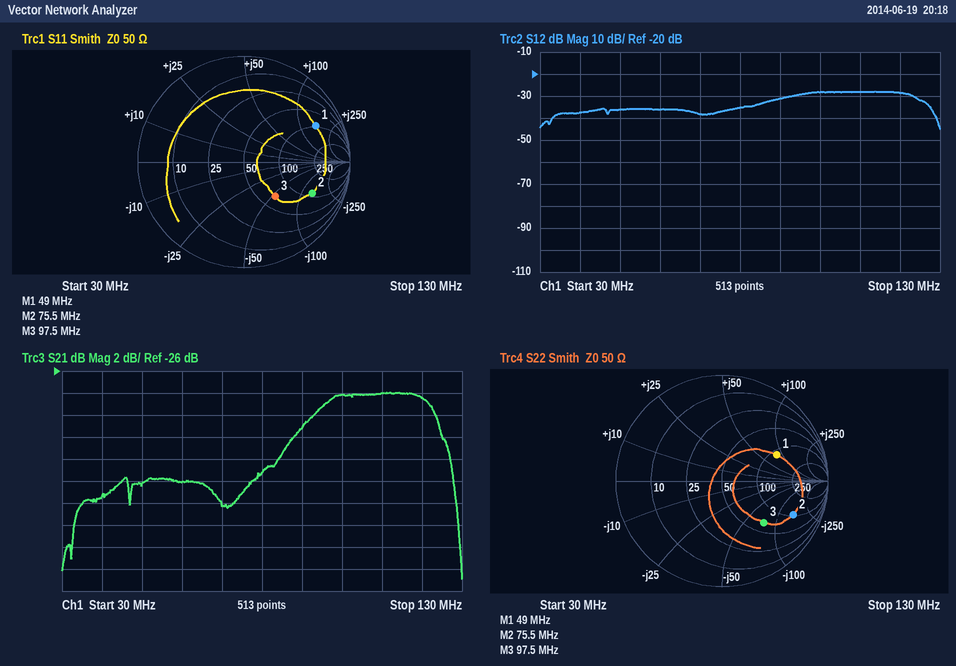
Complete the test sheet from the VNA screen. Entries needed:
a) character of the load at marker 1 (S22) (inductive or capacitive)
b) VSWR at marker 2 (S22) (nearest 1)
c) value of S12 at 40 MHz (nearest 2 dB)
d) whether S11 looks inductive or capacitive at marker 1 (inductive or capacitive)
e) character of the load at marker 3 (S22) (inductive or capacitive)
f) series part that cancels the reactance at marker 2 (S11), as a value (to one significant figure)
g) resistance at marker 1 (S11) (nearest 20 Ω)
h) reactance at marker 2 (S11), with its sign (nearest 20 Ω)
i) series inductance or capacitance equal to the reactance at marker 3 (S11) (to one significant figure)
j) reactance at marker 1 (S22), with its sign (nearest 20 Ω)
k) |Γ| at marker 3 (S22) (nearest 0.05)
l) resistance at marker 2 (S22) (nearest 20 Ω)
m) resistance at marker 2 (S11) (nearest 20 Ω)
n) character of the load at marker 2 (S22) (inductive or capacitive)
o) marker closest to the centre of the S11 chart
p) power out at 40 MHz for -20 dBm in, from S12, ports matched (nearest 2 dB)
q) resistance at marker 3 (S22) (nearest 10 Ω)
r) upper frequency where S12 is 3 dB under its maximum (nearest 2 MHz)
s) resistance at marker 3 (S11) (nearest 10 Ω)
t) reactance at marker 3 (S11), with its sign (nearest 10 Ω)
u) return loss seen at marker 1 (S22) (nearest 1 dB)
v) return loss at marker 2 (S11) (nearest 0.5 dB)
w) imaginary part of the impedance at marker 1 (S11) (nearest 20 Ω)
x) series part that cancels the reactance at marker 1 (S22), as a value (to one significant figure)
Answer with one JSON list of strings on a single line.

["inductive", "7", "-38 dB", "inductive", "capacitive", "300 nH", "100 Ω", "-140 Ω", "30 pF", "+80 Ω", "0.55", "100 Ω", "120 Ω", "capacitive", "marker 3", "-58 dBm", "70 Ω", "124 MHz", "70 Ω", "-50 Ω", "5 dB", "3.0 dB", "+160 Ω", "40 pF"]
